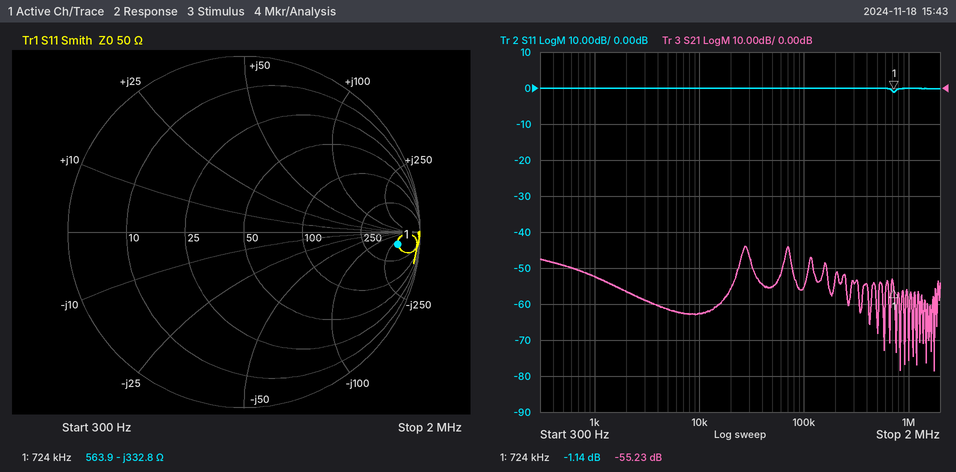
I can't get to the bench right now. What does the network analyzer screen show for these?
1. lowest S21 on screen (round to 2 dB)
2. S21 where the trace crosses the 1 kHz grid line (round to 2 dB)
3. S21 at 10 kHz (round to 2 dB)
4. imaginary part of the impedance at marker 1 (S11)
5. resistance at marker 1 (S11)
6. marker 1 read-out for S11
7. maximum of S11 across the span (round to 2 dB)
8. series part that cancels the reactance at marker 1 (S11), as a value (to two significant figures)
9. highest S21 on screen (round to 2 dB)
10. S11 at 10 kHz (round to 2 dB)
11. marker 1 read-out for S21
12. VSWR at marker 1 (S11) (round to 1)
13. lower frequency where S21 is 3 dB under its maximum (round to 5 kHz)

-78 dB
-52 dB
-62 dB
-332.8 Ω
563.9 Ω
-1.14 dB
0 dB
73 µH
-44 dB
0 dB
-55.23 dB
15
25 kHz
